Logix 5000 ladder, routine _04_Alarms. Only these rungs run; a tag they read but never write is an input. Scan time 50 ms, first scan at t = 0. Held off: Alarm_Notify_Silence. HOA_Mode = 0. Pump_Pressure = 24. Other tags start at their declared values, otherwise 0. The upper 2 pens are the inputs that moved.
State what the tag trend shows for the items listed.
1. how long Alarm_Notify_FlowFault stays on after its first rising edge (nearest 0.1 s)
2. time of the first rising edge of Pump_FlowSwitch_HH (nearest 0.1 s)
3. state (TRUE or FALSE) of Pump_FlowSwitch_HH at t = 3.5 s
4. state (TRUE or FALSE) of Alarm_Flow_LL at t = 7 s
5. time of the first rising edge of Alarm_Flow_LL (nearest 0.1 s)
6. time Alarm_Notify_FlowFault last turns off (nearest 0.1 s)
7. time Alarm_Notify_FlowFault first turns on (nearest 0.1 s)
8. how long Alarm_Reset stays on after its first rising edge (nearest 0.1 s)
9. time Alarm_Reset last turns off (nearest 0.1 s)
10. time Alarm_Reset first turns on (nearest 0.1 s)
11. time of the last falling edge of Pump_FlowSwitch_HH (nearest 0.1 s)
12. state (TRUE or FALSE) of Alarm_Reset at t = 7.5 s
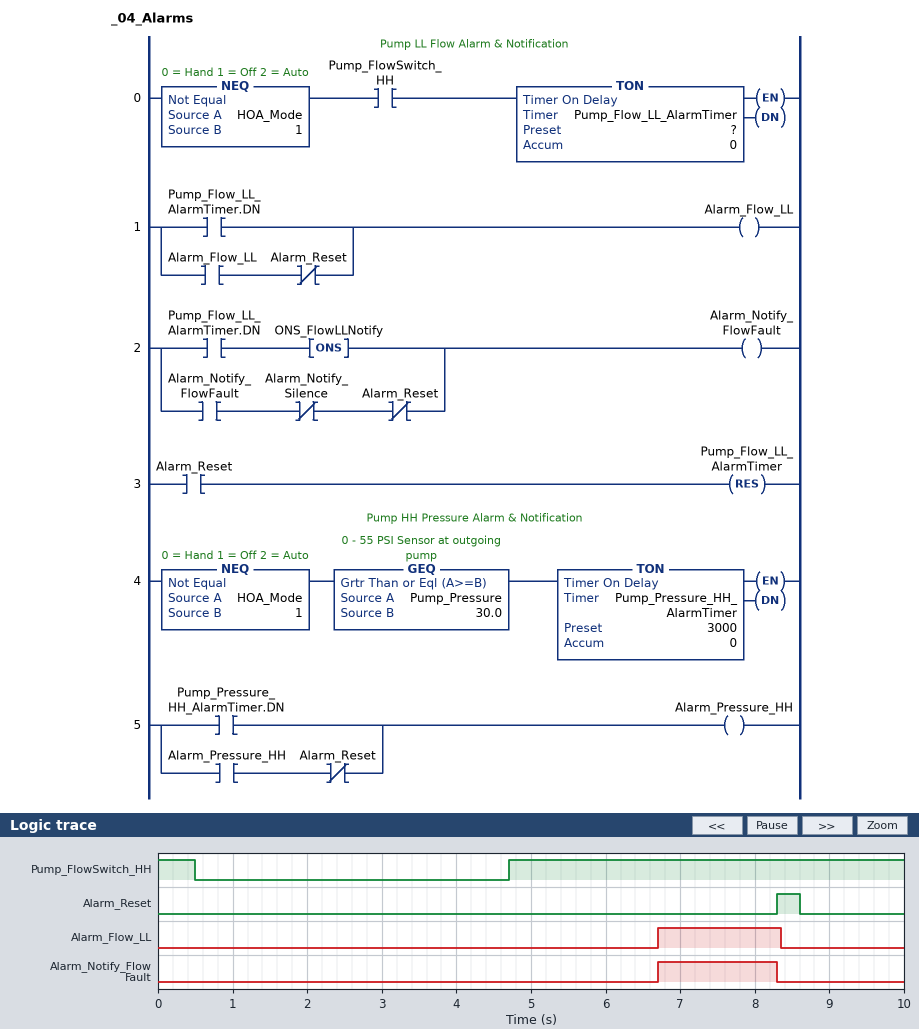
1.6 s
4.7 s
FALSE
TRUE
6.7 s
8.3 s
6.7 s
0.3 s
8.6 s
8.3 s
0.5 s
FALSE
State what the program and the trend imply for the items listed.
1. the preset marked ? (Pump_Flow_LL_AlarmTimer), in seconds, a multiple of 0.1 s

2.0 s
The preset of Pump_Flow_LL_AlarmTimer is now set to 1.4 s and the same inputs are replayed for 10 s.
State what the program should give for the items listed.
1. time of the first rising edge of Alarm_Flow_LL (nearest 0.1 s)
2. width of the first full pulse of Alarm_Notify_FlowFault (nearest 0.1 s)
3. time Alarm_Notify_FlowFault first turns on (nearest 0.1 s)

6.1 s
2.2 s
6.1 s
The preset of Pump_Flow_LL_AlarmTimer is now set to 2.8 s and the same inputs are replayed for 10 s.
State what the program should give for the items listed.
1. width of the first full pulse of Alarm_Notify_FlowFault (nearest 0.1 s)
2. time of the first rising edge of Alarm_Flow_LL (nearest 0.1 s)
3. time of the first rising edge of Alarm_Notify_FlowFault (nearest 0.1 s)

0.8 s
7.5 s
7.5 s
